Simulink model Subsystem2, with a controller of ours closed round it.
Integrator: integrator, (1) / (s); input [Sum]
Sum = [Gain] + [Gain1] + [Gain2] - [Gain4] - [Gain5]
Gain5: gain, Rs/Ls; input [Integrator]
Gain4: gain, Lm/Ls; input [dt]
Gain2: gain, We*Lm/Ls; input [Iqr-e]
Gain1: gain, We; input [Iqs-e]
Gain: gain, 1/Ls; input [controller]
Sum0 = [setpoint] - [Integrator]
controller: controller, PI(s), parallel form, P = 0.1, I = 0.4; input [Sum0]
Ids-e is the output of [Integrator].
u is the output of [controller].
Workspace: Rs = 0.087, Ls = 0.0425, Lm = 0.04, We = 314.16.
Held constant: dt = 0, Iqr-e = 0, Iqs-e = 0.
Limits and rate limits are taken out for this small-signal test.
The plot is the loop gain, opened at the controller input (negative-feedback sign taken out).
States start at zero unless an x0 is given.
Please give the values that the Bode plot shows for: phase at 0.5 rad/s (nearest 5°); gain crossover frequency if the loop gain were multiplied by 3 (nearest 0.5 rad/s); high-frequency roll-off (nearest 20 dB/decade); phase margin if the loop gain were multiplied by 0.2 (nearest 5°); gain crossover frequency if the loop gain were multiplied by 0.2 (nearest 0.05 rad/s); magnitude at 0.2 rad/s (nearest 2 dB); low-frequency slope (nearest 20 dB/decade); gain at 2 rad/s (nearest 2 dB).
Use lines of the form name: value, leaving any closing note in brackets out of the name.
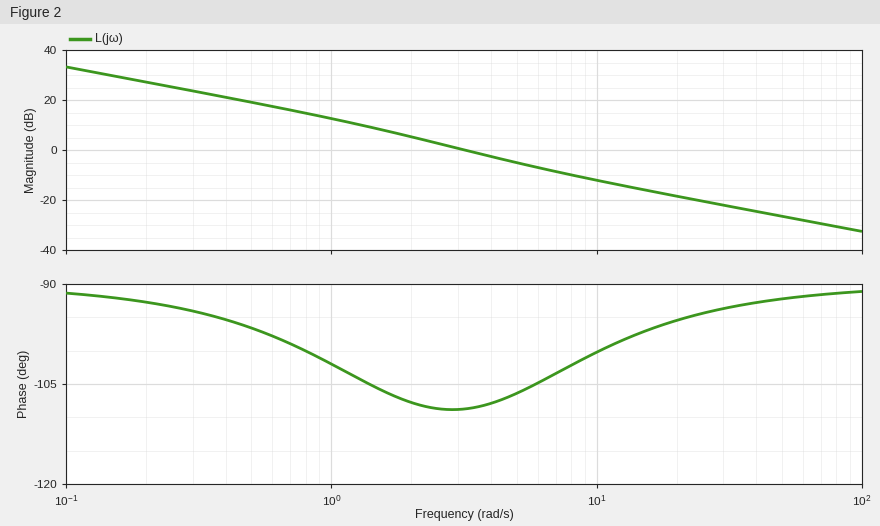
phase at 0.5 rad/s: -95°
gain crossover frequency if the loop gain were multiplied by 3: 7.5 rad/s
high-frequency roll-off: -20 dB/decade
phase margin if the loop gain were multiplied by 0.2: 80°
gain crossover frequency if the loop gain were multiplied by 0.2: 0.85 rad/s
magnitude at 0.2 rad/s: 28 dB
low-frequency slope: -20 dB/decade
gain at 2 rad/s: 6 dB
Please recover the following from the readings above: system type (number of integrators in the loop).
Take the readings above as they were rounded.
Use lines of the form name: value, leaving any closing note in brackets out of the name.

system type: 1
